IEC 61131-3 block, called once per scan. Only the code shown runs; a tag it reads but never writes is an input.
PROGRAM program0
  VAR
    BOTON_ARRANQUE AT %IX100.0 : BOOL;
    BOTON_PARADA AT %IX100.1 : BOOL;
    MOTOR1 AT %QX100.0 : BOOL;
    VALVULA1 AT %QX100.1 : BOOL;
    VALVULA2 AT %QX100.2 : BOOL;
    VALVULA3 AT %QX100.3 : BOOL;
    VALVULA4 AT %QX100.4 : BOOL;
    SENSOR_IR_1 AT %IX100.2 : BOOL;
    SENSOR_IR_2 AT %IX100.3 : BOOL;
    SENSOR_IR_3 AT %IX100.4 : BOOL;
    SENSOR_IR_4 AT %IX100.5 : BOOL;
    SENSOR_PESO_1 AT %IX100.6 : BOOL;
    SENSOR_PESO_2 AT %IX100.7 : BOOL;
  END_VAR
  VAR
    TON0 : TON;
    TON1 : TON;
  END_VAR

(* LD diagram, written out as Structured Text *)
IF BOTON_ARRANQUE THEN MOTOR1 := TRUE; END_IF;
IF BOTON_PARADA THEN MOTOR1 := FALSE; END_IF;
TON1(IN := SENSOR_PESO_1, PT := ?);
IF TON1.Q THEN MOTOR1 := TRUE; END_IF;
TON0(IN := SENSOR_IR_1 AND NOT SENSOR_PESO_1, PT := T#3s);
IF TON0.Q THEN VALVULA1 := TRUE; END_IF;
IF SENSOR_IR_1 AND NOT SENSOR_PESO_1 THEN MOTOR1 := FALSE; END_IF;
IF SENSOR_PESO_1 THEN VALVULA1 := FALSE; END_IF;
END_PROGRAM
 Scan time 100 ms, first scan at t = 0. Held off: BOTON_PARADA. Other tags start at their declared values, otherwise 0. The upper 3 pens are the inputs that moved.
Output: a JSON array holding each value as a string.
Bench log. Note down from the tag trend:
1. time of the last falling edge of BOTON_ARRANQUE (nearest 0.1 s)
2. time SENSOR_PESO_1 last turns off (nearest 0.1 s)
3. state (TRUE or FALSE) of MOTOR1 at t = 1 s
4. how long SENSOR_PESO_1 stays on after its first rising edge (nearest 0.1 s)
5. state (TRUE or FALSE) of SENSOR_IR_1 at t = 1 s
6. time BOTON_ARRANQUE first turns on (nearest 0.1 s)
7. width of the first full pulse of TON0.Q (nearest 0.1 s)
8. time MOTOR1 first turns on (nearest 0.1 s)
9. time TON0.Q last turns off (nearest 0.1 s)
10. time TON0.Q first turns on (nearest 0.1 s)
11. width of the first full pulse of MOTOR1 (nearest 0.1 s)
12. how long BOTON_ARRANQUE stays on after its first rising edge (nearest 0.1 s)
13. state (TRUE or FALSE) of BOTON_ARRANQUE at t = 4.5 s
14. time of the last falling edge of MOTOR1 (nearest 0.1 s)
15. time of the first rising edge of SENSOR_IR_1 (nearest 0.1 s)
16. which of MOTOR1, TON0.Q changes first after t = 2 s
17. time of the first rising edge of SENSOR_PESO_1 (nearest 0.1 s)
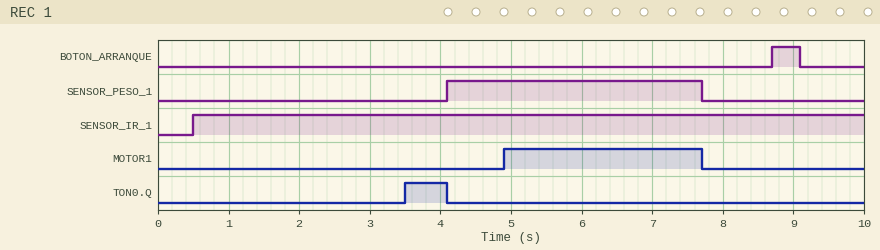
["9.1 s", "7.7 s", "FALSE", "3.6 s", "TRUE", "8.7 s", "0.6 s", "4.9 s", "4.1 s", "3.5 s", "2.8 s", "0.4 s", "FALSE", "7.7 s", "0.5 s", "TON0.Q", "4.1 s"]
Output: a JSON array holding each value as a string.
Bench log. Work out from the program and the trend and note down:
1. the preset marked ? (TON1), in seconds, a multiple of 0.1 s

["0.8 s"]
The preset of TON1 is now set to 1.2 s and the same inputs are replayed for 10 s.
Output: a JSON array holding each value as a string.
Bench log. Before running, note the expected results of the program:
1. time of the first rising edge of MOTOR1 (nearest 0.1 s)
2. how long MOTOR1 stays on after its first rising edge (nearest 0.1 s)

["5.3 s", "2.4 s"]
